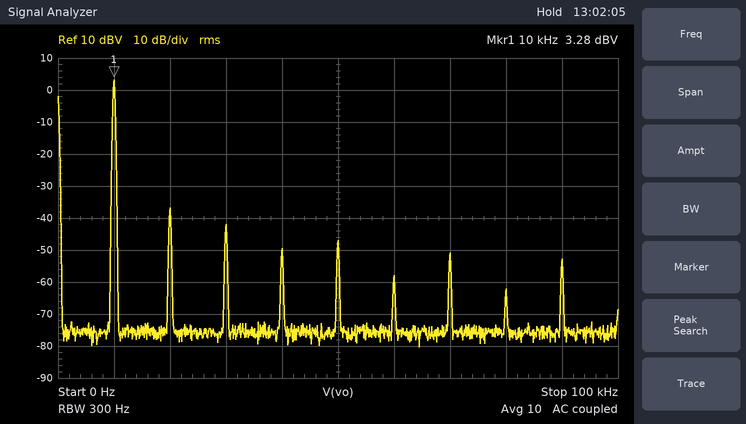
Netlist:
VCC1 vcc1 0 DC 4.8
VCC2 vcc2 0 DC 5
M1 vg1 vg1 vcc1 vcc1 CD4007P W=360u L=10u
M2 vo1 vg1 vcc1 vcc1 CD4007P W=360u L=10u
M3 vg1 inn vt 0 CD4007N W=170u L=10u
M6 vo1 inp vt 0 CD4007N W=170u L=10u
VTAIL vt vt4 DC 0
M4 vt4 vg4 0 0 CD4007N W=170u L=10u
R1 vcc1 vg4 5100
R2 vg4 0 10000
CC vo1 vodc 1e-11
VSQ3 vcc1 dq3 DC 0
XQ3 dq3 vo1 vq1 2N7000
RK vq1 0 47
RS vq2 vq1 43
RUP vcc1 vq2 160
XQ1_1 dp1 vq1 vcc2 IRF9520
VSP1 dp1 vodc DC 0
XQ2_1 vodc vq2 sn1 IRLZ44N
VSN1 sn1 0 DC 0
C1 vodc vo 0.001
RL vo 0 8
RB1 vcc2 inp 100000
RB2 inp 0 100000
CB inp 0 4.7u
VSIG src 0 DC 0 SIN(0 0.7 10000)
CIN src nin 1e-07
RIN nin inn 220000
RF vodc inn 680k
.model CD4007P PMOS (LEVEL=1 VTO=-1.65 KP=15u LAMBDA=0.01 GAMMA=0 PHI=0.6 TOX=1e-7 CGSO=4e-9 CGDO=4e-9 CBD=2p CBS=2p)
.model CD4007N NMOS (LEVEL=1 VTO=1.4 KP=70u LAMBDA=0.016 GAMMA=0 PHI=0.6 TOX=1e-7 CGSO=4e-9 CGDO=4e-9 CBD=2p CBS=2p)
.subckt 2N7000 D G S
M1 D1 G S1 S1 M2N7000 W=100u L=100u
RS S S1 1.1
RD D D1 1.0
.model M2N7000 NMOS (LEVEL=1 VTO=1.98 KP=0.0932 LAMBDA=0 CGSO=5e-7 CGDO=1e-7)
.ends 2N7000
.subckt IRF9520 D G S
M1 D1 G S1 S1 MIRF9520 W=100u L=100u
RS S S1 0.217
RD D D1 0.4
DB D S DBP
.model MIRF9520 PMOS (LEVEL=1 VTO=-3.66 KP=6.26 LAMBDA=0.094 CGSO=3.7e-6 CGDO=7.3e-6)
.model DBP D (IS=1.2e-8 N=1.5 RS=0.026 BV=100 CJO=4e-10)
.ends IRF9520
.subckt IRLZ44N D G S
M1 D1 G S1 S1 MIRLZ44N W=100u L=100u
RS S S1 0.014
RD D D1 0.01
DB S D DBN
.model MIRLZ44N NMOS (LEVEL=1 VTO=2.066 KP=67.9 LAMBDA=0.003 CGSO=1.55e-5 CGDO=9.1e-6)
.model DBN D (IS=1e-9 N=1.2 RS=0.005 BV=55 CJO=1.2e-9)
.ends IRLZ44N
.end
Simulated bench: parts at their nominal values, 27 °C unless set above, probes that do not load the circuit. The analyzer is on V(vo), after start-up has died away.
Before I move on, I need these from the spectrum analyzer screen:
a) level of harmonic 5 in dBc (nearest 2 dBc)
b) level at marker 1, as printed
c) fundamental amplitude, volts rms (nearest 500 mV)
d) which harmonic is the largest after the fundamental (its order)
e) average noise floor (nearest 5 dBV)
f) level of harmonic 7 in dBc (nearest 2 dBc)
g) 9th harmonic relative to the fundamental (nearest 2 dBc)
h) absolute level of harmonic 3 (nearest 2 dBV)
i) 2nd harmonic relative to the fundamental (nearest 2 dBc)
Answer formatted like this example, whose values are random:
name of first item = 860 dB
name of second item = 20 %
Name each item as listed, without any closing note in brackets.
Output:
level of harmonic 5 in dBc = -50 dBc
level at marker 1, as printed = 3.28 dBV
fundamental amplitude, volts rms = 1.5 V
which harmonic is the largest after the fundamental = 2
average noise floor = -75 dBV
level of harmonic 7 in dBc = -54 dBc
9th harmonic relative to the fundamental = -56 dBc
absolute level of harmonic 3 = -42 dBV
2nd harmonic relative to the fundamental = -40 dBc
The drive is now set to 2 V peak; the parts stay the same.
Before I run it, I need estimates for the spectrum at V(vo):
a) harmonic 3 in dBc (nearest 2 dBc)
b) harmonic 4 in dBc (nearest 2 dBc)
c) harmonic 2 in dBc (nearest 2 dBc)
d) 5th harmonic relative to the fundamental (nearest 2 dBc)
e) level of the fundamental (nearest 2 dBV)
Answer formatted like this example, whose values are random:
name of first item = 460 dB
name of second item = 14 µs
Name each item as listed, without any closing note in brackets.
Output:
harmonic 3 in dBc = -12 dBc
harmonic 4 in dBc = -32 dBc
harmonic 2 in dBc = -28 dBc
5th harmonic relative to the fundamental = -20 dBc
level of the fundamental = 6 dBV
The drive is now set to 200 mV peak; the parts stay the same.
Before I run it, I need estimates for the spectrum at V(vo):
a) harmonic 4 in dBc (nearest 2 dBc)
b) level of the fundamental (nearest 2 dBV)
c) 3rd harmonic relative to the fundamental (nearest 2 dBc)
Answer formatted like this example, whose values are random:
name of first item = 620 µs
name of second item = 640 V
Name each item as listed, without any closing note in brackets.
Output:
harmonic 4 in dBc = -58 dBc
level of the fundamental = -8 dBV
3rd harmonic relative to the fundamental = -36 dBc
